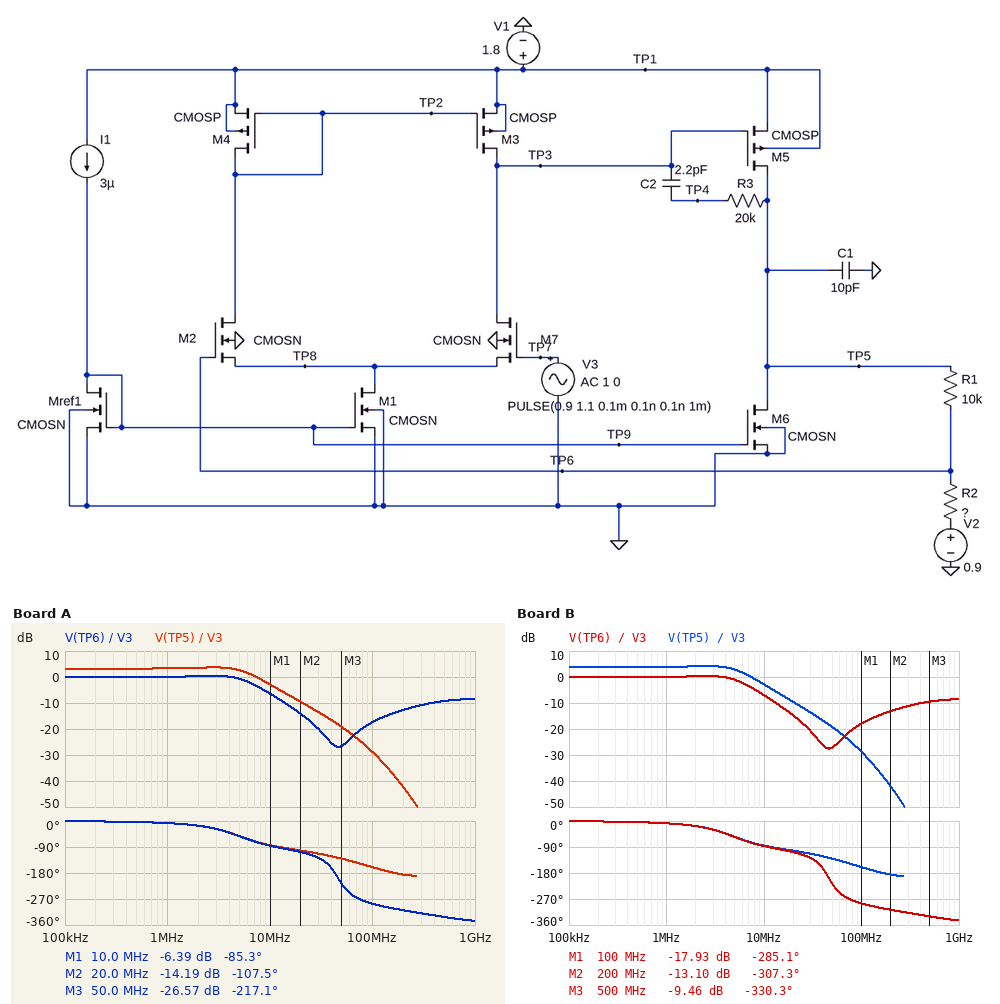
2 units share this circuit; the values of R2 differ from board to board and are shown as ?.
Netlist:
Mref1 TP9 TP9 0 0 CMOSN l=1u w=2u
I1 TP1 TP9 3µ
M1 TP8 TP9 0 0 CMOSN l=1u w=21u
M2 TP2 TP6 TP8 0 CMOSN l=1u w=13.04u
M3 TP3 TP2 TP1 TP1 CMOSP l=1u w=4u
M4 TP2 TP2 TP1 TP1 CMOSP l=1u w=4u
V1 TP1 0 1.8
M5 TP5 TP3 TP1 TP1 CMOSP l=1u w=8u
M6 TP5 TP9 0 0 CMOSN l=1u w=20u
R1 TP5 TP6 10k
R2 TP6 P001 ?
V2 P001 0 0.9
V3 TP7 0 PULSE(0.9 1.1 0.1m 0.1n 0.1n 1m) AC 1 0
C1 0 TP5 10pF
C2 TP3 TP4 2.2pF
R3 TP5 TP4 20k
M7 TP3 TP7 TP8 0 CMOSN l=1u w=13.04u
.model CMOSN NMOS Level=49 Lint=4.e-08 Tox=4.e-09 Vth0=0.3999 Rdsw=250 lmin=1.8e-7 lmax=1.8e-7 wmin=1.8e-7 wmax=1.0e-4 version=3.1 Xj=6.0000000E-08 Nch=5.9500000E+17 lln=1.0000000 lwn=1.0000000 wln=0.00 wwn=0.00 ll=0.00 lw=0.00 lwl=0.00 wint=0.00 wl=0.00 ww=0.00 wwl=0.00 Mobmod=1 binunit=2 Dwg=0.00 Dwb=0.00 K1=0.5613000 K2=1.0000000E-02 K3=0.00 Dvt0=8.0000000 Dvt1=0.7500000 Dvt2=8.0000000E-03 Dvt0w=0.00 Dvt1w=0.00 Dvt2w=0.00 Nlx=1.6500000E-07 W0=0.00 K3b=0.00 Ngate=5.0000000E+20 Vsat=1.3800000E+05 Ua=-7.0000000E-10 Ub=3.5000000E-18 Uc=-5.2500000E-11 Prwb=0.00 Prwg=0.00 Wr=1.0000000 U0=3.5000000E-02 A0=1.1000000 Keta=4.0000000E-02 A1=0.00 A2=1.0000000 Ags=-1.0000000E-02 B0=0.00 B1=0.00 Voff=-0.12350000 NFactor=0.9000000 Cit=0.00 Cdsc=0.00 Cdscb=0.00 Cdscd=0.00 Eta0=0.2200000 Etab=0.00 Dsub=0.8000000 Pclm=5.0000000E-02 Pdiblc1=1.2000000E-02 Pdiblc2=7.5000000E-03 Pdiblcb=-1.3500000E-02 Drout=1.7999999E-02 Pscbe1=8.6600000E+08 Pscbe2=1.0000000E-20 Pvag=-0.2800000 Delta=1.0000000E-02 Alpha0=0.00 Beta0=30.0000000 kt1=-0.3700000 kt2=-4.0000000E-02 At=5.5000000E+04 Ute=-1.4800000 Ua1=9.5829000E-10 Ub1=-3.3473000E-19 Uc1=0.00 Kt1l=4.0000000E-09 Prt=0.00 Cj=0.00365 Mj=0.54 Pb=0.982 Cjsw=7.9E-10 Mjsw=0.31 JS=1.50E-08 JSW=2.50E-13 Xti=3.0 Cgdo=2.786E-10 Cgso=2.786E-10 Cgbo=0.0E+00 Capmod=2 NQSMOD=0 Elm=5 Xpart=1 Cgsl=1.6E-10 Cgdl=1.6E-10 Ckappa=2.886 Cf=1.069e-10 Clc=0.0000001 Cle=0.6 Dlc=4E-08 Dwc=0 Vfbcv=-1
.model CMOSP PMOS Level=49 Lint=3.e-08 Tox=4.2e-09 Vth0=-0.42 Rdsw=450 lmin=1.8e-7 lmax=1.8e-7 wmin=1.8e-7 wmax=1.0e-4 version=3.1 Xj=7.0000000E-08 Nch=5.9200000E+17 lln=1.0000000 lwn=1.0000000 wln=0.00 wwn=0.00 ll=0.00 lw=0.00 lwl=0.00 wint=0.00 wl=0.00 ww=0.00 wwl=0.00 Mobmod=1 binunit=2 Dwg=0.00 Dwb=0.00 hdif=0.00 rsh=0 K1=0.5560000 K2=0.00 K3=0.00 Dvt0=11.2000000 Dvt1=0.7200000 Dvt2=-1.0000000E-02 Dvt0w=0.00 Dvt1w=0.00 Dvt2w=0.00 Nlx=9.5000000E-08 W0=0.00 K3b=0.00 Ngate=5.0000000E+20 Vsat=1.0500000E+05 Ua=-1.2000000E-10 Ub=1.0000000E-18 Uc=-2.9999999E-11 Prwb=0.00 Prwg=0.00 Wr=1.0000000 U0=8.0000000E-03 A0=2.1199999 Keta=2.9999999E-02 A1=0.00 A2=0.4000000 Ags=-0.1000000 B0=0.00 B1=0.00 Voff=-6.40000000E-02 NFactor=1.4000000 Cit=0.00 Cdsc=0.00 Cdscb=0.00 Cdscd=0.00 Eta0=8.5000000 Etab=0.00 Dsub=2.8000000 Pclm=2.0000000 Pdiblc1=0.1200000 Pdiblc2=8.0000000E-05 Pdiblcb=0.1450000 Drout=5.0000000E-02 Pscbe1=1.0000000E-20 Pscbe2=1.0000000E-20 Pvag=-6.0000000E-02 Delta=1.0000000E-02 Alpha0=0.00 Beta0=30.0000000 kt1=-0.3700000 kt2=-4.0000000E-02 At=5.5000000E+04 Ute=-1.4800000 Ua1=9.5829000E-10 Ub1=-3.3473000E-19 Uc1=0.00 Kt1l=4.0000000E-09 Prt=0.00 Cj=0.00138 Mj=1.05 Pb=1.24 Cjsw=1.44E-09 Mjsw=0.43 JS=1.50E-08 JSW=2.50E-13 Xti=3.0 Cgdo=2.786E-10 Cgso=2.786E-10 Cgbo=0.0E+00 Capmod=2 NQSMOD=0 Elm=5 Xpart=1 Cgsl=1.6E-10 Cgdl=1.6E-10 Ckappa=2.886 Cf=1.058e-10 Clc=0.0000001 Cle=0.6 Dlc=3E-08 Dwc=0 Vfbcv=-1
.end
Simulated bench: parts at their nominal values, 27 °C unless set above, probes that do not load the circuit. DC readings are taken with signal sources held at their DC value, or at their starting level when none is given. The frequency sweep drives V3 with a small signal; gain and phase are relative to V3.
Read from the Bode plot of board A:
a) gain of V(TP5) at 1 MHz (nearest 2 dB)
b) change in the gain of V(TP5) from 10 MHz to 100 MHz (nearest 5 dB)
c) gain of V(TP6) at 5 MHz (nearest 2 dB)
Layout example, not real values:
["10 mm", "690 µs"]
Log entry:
["4 dB", "-25 dB", "0 dB"]
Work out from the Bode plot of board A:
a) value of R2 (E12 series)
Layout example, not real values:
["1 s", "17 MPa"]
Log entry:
["22 kΩ"]
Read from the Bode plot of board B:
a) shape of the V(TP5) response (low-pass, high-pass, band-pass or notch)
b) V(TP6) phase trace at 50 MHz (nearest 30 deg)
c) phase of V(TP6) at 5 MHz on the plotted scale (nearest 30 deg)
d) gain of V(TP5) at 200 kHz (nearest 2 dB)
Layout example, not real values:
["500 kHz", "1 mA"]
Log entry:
["low-pass", "-210 deg", "-60 deg", "4 dB"]
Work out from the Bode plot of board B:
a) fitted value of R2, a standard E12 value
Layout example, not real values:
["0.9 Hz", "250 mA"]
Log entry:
["18 kΩ"]
